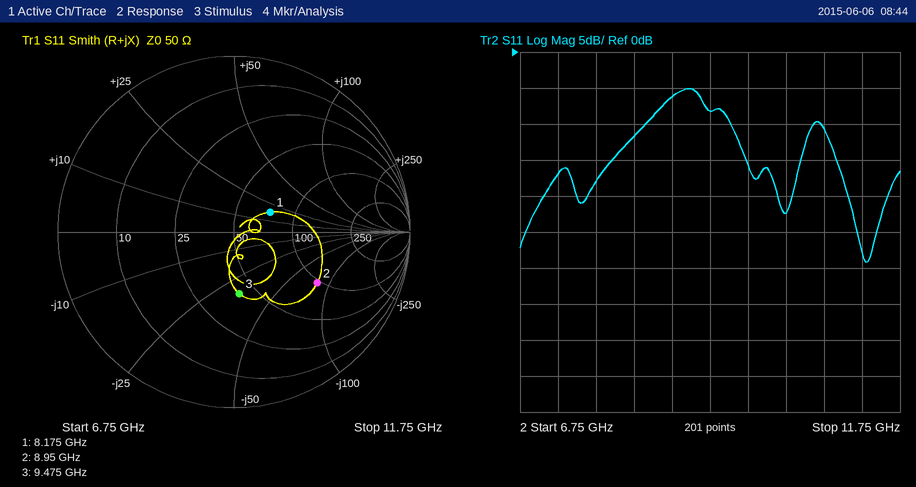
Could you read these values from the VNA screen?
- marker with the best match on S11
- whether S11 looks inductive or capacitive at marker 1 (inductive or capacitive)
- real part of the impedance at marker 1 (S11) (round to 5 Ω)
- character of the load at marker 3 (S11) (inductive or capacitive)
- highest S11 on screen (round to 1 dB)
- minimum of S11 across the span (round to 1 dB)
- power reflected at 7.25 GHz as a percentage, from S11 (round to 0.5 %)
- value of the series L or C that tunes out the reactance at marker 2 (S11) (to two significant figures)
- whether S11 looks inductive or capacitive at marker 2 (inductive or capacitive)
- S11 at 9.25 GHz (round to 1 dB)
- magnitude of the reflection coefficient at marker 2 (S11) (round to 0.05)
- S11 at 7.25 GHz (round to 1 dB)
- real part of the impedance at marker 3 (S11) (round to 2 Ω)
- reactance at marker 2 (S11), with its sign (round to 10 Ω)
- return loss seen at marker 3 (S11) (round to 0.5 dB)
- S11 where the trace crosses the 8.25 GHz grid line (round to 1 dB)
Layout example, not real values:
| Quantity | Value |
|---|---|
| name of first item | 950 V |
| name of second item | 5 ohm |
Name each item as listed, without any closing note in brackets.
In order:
| Quantity | Value |
|---|---|
| marker with the best match on S11 | marker 1 |
| whether S11 looks inductive or capacitive at marker 1 | inductive |
| real part of the impedance at marker 1 (S11) | 75 Ω |
| character of the load at marker 3 (S11) | capacitive |
| highest S11 on screen | -5 dB |
| minimum of S11 across the span | -29 dB |
| power reflected at 7.25 GHz as a percentage, from S11 | 2.0 % |
| value of the series L or C that tunes out the reactance at marker 2 (S11) | 1.4 nH |
| whether S11 looks inductive or capacitive at marker 2 | capacitive |
| S11 at 9.25 GHz | -8 dB |
| magnitude of the reflection coefficient at marker 2 (S11) | 0.55 |
| S11 at 7.25 GHz | -17 dB |
| real part of the impedance at marker 3 (S11) | 42 Ω |
| reactance at marker 2 (S11), with its sign | -80 Ω |
| return loss seen at marker 3 (S11) | 9.0 dB |
| S11 where the trace crosses the 8.25 GHz grid line | -12 dB |
